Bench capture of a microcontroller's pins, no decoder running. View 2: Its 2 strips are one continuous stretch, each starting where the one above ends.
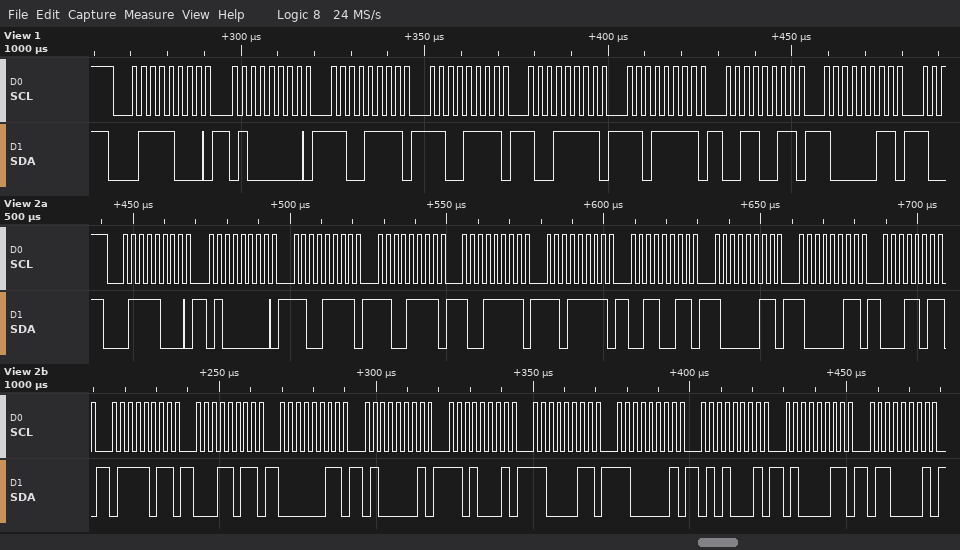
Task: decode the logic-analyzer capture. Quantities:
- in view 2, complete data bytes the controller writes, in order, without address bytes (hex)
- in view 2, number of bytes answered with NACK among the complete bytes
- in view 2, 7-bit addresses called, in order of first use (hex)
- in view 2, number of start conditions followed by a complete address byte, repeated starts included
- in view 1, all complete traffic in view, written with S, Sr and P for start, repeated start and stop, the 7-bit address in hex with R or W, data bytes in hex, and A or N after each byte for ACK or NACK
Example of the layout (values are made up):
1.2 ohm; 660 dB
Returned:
40 CF CF 9F DF 33 83 83 1B 7B 1B 03 41 D1 C3 C1 51 43 61; 0; 0x3C; 1; S 3CW A 40 A CF A CF A 9F A DF A 33 A 83 A
